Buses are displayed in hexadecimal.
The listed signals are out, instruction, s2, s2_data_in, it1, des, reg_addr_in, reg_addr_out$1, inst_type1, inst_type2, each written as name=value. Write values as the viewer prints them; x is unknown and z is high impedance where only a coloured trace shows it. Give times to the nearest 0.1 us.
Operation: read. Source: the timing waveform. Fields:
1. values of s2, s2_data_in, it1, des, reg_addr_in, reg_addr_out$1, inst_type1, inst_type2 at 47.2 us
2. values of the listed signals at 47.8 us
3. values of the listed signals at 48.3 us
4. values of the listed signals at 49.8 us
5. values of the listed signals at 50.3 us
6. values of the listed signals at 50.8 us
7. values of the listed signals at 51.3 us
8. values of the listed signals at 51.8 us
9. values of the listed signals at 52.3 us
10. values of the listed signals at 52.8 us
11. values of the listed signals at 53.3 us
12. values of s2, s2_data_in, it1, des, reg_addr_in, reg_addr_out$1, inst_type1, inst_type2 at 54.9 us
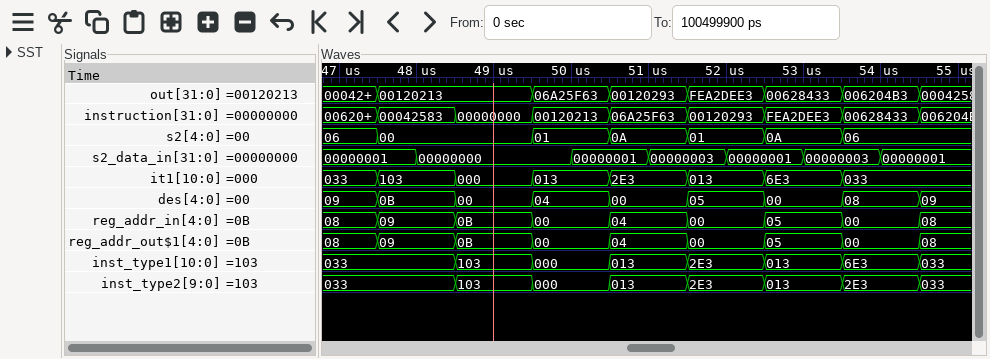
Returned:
s2=06, s2_data_in=00000001, it1=033, des=09, reg_addr_in=08, reg_addr_out$1=08, inst_type1=033, inst_type2=033
out=00120213, instruction=00042583, s2=00, s2_data_in=00000001, it1=103, des=0B, reg_addr_in=09, reg_addr_out$1=09, inst_type1=033, inst_type2=033
out=00120213, instruction=00042583, s2=00, s2_data_in=00000000, it1=103, des=0B, reg_addr_in=09, reg_addr_out$1=09, inst_type1=033, inst_type2=033
out=06A25F63, instruction=00120213, s2=01, s2_data_in=00000000, it1=013, des=04, reg_addr_in=00, reg_addr_out$1=00, inst_type1=000, inst_type2=000
out=06A25F63, instruction=00120213, s2=01, s2_data_in=00000001, it1=013, des=04, reg_addr_in=00, reg_addr_out$1=00, inst_type1=000, inst_type2=000
out=00120293, instruction=06A25F63, s2=0A, s2_data_in=00000001, it1=2E3, des=00, reg_addr_in=04, reg_addr_out$1=04, inst_type1=013, inst_type2=013
out=00120293, instruction=06A25F63, s2=0A, s2_data_in=00000003, it1=2E3, des=00, reg_addr_in=04, reg_addr_out$1=04, inst_type1=013, inst_type2=013
out=FEA2DEE3, instruction=00120293, s2=01, s2_data_in=00000003, it1=013, des=05, reg_addr_in=00, reg_addr_out$1=00, inst_type1=2E3, inst_type2=2E3
out=FEA2DEE3, instruction=00120293, s2=01, s2_data_in=00000001, it1=013, des=05, reg_addr_in=00, reg_addr_out$1=00, inst_type1=2E3, inst_type2=2E3
out=00628433, instruction=FEA2DEE3, s2=0A, s2_data_in=00000001, it1=6E3, des=00, reg_addr_in=05, reg_addr_out$1=05, inst_type1=013, inst_type2=013
out=00628433, instruction=FEA2DEE3, s2=0A, s2_data_in=00000003, it1=6E3, des=00, reg_addr_in=05, reg_addr_out$1=05, inst_type1=013, inst_type2=013
s2=06, s2_data_in=00000001, it1=033, des=09, reg_addr_in=08, reg_addr_out$1=08, inst_type1=033, inst_type2=033
